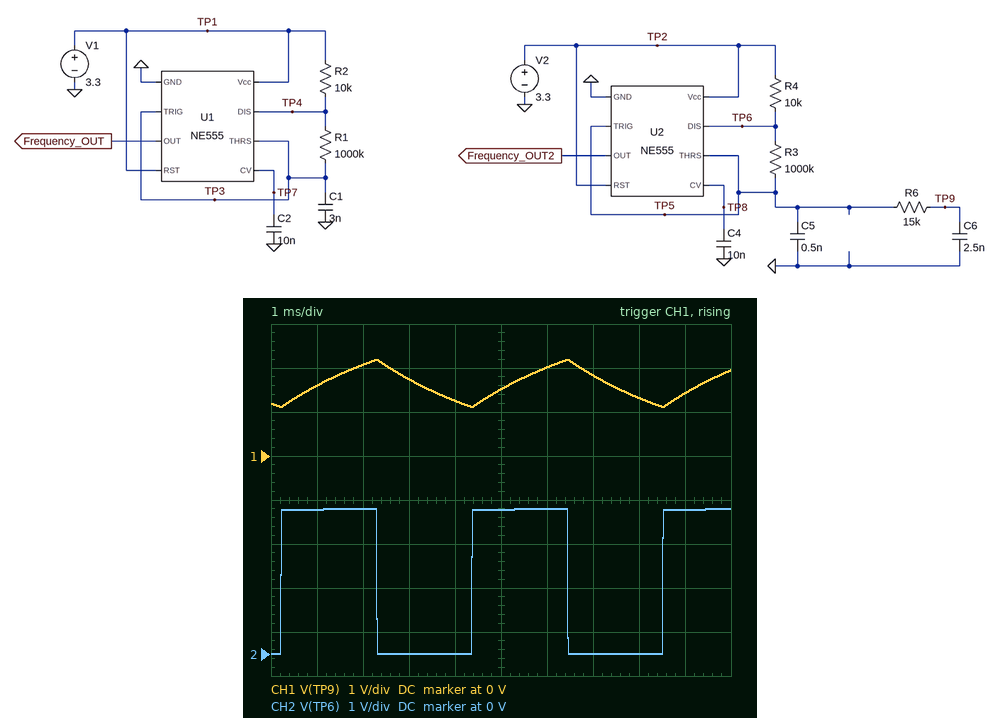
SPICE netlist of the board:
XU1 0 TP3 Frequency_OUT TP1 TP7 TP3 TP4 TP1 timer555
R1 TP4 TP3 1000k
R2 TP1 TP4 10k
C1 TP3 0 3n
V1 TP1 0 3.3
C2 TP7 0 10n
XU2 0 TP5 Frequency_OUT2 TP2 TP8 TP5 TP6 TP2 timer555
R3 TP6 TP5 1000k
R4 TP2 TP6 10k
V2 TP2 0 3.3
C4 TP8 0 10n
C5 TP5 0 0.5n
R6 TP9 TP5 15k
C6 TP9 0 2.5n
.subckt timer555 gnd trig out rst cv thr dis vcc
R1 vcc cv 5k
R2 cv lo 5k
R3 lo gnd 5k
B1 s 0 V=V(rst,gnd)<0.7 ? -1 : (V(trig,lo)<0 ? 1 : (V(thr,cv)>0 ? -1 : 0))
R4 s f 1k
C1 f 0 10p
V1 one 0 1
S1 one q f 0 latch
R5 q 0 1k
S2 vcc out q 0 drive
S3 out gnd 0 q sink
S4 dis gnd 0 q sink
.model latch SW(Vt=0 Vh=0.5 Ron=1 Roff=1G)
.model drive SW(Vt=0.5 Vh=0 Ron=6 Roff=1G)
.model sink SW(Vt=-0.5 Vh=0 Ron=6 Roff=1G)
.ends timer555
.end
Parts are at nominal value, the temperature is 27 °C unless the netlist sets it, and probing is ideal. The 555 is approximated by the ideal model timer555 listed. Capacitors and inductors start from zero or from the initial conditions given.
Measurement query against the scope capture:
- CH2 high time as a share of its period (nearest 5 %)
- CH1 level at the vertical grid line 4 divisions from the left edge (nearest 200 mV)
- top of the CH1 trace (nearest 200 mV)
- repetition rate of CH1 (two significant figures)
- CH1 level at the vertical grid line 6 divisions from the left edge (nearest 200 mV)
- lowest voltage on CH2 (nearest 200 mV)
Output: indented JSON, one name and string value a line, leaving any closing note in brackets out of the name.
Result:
{
  "CH2 high time as a share of its period": "50 %",
  "CH1 level at the vertical grid line 4 divisions from the left edge": "1.2 V",
  "top of the CH1 trace": "2.2 V",
  "repetition rate of CH1": "240 Hz",
  "CH1 level at the vertical grid line 6 divisions from the left edge": "2.0 V",
  "lowest voltage on CH2": "0 V"
}
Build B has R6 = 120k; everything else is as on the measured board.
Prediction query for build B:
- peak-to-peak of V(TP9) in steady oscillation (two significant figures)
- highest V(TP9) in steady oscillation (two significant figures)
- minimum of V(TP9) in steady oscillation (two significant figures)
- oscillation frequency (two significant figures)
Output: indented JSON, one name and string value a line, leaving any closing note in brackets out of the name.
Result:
{
  "peak-to-peak of V(TP9) in steady oscillation": "890 mV",
  "highest V(TP9) in steady oscillation": "2.1 V",
  "minimum of V(TP9) in steady oscillation": "1.2 V",
  "oscillation frequency": "270 Hz"
}
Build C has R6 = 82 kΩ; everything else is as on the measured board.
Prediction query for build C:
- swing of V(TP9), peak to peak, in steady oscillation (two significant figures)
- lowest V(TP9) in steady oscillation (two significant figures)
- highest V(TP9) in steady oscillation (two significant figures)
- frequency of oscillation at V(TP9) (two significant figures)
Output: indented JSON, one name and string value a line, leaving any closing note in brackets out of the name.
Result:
{
  "swing of V(TP9), peak to peak, in steady oscillation": "950 mV",
  "lowest V(TP9) in steady oscillation": "1.2 V",
  "highest V(TP9) in steady oscillation": "2.1 V",
  "frequency of oscillation at V(TP9)": "260 Hz"
}
